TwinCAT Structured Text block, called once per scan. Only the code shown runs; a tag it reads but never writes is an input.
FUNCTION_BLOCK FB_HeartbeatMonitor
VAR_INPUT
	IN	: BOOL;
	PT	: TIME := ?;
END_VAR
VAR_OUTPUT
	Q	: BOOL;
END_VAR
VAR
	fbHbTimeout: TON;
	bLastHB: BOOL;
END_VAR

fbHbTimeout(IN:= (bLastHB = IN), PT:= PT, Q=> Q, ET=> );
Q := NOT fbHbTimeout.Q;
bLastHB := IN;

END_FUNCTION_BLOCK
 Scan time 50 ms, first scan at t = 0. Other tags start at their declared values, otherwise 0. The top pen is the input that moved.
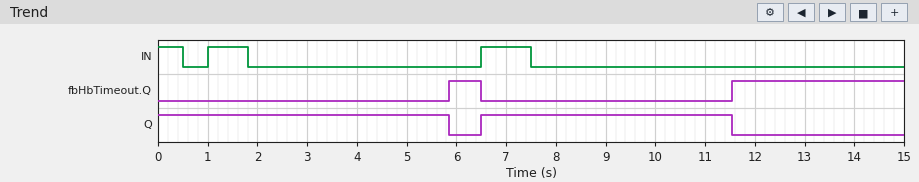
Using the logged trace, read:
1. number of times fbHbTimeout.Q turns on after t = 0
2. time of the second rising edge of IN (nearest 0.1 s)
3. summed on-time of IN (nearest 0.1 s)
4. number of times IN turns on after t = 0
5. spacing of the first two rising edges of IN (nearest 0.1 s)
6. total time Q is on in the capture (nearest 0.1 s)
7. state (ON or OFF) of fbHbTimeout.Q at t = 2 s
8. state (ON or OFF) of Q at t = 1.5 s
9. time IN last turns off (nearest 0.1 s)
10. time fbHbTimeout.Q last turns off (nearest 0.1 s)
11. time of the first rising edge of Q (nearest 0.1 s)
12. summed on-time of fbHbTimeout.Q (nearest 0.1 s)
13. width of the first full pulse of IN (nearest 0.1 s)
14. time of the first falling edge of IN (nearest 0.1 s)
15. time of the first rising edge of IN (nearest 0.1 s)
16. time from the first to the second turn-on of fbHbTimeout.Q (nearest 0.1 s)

2
6.5 s
2.3 s
2
5.5 s
10.9 s
OFF
ON
7.5 s
6.5 s
6.5 s
4.1 s
0.8 s
0.5 s
1.0 s
5.7 s
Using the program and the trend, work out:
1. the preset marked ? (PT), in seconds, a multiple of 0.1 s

4.0 s
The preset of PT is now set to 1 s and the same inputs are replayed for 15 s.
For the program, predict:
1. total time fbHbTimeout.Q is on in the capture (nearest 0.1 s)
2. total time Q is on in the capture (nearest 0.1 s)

10.1 s
4.9 s
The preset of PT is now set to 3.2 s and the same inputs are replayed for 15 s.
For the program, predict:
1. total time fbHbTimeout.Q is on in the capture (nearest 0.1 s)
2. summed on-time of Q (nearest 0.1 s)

5.7 s
9.3 s
